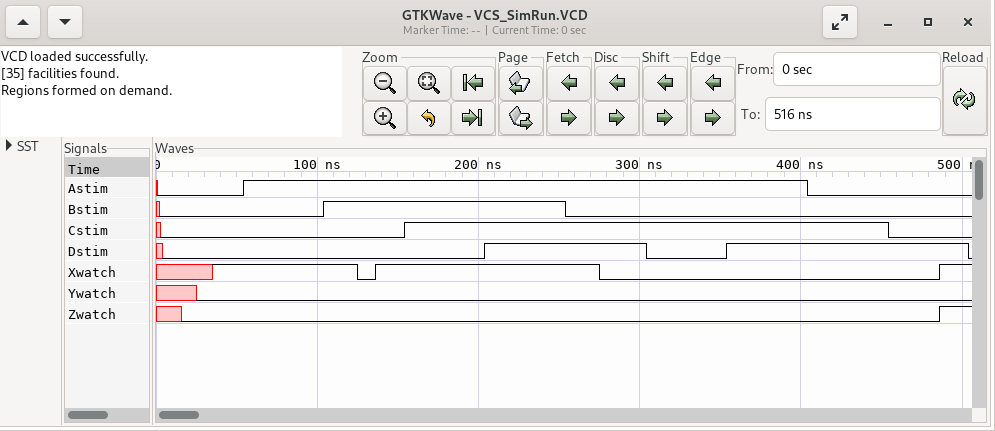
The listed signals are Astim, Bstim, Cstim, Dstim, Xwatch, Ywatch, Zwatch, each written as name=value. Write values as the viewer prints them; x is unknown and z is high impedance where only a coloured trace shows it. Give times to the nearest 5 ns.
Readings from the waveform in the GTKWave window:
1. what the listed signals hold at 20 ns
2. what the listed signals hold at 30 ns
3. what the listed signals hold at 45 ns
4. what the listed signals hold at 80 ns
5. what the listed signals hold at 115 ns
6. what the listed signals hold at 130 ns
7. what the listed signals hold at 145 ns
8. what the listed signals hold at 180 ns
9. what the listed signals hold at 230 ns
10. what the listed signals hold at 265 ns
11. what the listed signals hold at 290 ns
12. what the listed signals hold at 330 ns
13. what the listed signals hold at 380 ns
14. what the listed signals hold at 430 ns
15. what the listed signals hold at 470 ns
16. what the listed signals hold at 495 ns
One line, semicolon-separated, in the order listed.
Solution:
Astim=0, Bstim=0, Cstim=0, Dstim=0, Xwatch=x, Ywatch=x, Zwatch=0; Astim=0, Bstim=0, Cstim=0, Dstim=0, Xwatch=x, Ywatch=0, Zwatch=0; Astim=0, Bstim=0, Cstim=0, Dstim=0, Xwatch=1, Ywatch=0, Zwatch=0; Astim=1, Bstim=0, Cstim=0, Dstim=0, Xwatch=1, Ywatch=0, Zwatch=0; Astim=1, Bstim=1, Cstim=0, Dstim=0, Xwatch=1, Ywatch=0, Zwatch=0; Astim=1, Bstim=1, Cstim=0, Dstim=0, Xwatch=0, Ywatch=0, Zwatch=0; Astim=1, Bstim=1, Cstim=0, Dstim=0, Xwatch=1, Ywatch=0, Zwatch=0; Astim=1, Bstim=1, Cstim=1, Dstim=0, Xwatch=1, Ywatch=0, Zwatch=0; Astim=1, Bstim=1, Cstim=1, Dstim=1, Xwatch=1, Ywatch=0, Zwatch=0; Astim=1, Bstim=0, Cstim=1, Dstim=1, Xwatch=1, Ywatch=0, Zwatch=0; Astim=1, Bstim=0, Cstim=1, Dstim=1, Xwatch=0, Ywatch=0, Zwatch=0; Astim=1, Bstim=0, Cstim=1, Dstim=0, Xwatch=0, Ywatch=0, Zwatch=0; Astim=1, Bstim=0, Cstim=1, Dstim=1, Xwatch=0, Ywatch=0, Zwatch=0; Astim=0, Bstim=0, Cstim=1, Dstim=1, Xwatch=0, Ywatch=0, Zwatch=0; Astim=0, Bstim=0, Cstim=0, Dstim=1, Xwatch=0, Ywatch=0, Zwatch=0; Astim=0, Bstim=0, Cstim=0, Dstim=1, Xwatch=1, Ywatch=0, Zwatch=1
